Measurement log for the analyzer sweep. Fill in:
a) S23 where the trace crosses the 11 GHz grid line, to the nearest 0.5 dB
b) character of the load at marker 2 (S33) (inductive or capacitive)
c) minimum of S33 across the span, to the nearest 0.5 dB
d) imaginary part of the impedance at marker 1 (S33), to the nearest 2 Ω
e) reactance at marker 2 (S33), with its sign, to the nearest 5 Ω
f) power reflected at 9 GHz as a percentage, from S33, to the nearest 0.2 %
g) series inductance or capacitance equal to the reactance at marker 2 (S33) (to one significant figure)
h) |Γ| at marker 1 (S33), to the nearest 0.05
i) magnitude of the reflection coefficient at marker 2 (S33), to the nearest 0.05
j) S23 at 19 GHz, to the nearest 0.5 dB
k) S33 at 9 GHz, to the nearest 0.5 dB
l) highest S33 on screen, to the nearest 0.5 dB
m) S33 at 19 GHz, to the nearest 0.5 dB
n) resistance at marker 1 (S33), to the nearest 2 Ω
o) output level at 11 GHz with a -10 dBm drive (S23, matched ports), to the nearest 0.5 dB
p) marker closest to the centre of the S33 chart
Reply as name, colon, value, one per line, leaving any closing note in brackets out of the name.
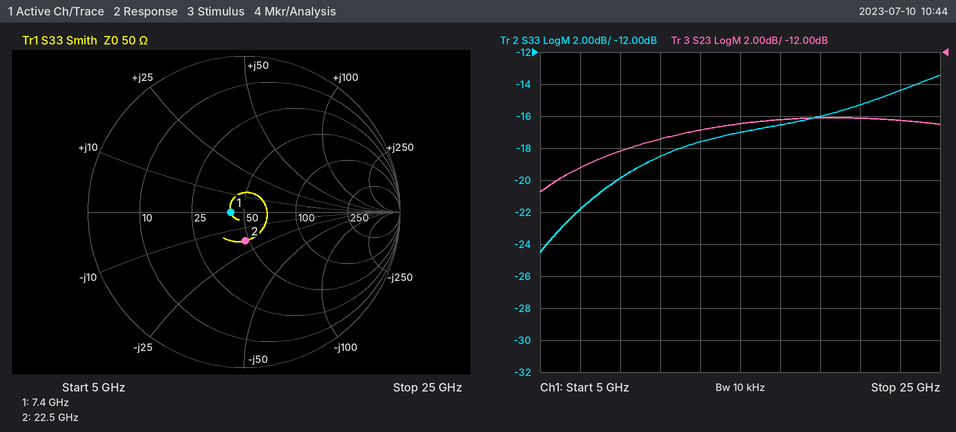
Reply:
S23 where the trace crosses the 11 GHz grid line, to the nearest 0.5 dB: -17.5 dB
character of the load at marker 2 (S33): capacitive
minimum of S33 across the span, to the nearest 0.5 dB: -24.5 dB
imaginary part of the impedance at marker 1 (S33), to the nearest 2 Ω: 0 Ω
reactance at marker 2 (S33), with its sign, to the nearest 5 Ω: -20 Ω
power reflected at 9 GHz as a percentage, from S33, to the nearest 0.2 %: 1.0 %
series inductance or capacitance equal to the reactance at marker 2 (S33): 400 fF
|Γ| at marker 1 (S33), to the nearest 0.05: 0.10
magnitude of the reflection coefficient at marker 2 (S33), to the nearest 0.05: 0.20
S23 at 19 GHz, to the nearest 0.5 dB: -16.0 dB
S33 at 9 GHz, to the nearest 0.5 dB: -20.0 dB
highest S33 on screen, to the nearest 0.5 dB: -13.5 dB
S33 at 19 GHz, to the nearest 0.5 dB: -16.0 dB
resistance at marker 1 (S33), to the nearest 2 Ω: 42 Ω
output level at 11 GHz with a -10 dBm drive (S23, matched ports), to the nearest 0.5 dB: -27.5 dBm
marker closest to the centre of the S33 chart: marker 1
